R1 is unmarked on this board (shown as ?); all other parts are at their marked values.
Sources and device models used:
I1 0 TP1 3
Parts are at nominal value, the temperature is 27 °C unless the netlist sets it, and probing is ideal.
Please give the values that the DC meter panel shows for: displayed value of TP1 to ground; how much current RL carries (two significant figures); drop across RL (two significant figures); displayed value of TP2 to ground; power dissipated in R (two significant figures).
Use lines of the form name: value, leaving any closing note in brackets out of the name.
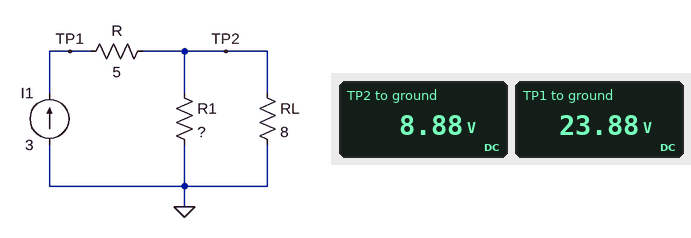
displayed value of TP1 to ground: 23.88 V
how much current RL carries: 1.1 A
drop across RL: 8.9 V
displayed value of TP2 to ground: 8.88 V
power dissipated in R: 45 W
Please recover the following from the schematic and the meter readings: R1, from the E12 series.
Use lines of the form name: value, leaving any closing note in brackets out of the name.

R1, from the E12 series: 4.7 Ω
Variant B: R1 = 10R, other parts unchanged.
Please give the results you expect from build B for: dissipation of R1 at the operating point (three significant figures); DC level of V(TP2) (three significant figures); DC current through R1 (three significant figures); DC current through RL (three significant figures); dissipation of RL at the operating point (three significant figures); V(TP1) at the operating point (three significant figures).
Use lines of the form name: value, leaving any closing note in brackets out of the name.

dissipation of R1 at the operating point: 17.8 W
DC level of V(TP2): 13.3 V
DC current through R1: 1.33 A
DC current through RL: 1.67 A
dissipation of RL at the operating point: 22.2 W
V(TP1) at the operating point: 28.3 V
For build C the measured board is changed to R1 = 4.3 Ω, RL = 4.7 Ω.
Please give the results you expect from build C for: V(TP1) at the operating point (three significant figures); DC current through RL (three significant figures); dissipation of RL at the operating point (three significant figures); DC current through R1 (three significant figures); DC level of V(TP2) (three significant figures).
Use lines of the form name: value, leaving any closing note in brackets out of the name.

V(TP1) at the operating point: 21.7 V
DC current through RL: 1.43 A
dissipation of RL at the operating point: 9.66 W
DC current through R1: 1.57 A
DC level of V(TP2): 6.74 V
